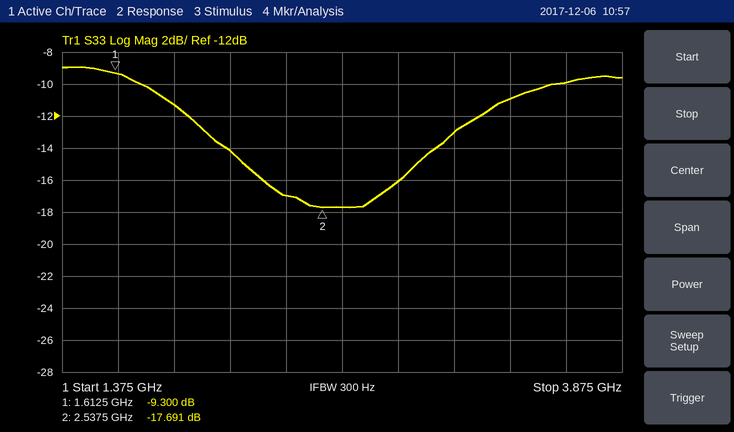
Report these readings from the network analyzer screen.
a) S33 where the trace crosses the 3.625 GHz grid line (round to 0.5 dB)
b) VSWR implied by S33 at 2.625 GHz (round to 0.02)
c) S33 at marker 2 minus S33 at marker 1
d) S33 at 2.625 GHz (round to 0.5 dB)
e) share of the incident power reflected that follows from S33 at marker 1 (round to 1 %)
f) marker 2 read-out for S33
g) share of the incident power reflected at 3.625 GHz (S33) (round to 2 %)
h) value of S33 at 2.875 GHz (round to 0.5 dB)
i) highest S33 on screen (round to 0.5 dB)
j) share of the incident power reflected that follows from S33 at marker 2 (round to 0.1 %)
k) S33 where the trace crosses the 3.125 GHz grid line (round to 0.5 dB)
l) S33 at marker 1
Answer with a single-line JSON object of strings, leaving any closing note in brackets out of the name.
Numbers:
{"S33 where the trace crosses the 3.625 GHz grid line": "-10.0 dB", "VSWR implied by S33 at 2.625 GHz": "1.30", "S33 at marker 2 minus S33 at marker 1": "-8.391 dB", "S33 at 2.625 GHz": "-17.5 dB", "share of the incident power reflected that follows from S33 at marker 1": "12 %", "marker 2 read-out for S33": "-17.691 dB", "share of the incident power reflected at 3.625 GHz (S33)": "10 %", "value of S33 at 2.875 GHz": "-16.0 dB", "highest S33 on screen": "-9.0 dB", "share of the incident power reflected that follows from S33 at marker 2": "1.7 %", "S33 where the trace crosses the 3.125 GHz grid line": "-13.0 dB", "S33 at marker 1": "-9.300 dB"}
